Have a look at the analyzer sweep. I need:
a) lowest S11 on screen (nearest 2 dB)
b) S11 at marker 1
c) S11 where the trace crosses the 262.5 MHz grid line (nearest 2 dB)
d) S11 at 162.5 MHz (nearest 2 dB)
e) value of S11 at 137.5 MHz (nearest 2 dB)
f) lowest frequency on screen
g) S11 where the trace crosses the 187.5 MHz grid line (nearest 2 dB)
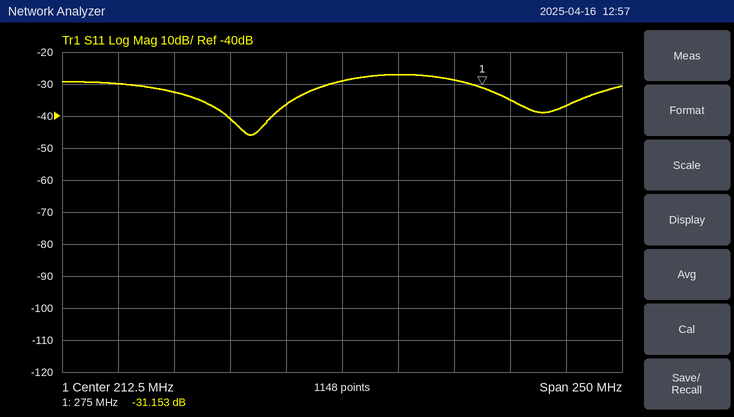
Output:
-46 dB
-31.153 dB
-28 dB
-40 dB
-32 dB
87.5 MHz
-36 dB
